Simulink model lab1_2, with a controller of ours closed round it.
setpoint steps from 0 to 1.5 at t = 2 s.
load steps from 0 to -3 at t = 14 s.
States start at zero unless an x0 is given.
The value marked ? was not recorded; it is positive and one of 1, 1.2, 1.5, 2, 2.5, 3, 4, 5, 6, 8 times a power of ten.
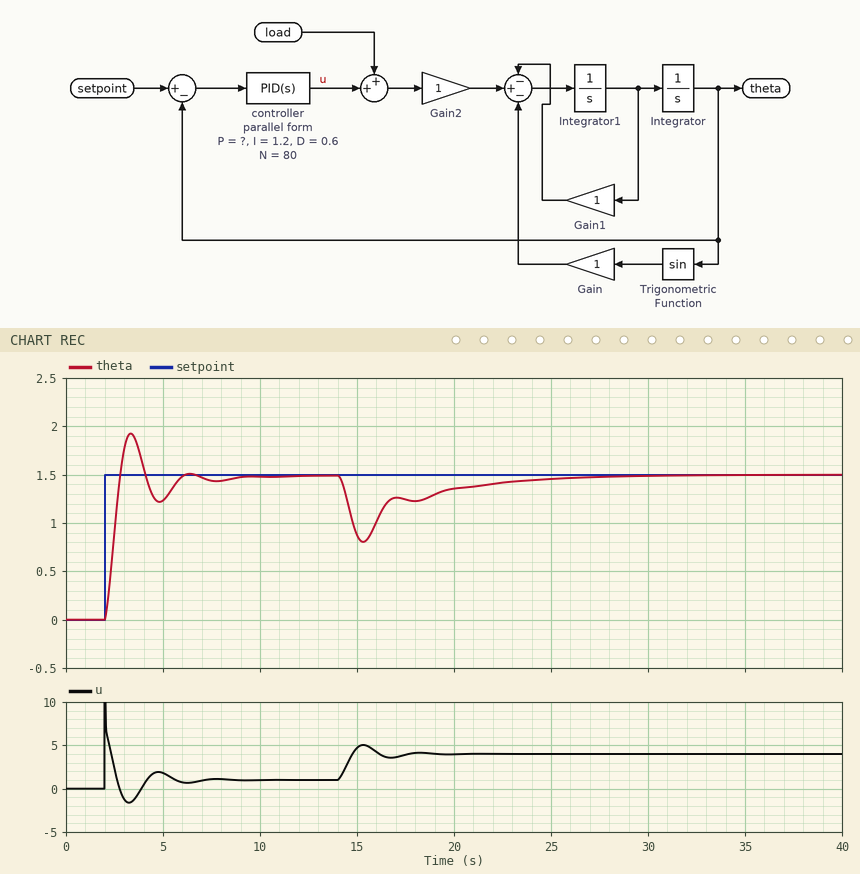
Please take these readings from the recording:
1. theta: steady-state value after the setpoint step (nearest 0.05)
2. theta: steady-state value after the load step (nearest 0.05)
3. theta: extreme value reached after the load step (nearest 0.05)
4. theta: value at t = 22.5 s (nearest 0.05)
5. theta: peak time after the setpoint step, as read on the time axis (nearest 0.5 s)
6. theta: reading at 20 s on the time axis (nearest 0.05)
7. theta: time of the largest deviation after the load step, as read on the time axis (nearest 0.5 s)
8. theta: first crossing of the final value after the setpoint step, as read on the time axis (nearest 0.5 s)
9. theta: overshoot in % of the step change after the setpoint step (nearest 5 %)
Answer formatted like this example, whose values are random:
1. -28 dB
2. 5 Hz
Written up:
1. 1.50
2. 1.50
3. 0.80
4. 1.40
5. 3.5 s
6. 1.35
7. 15.5 s
8. 3.0 s
9. 30 %
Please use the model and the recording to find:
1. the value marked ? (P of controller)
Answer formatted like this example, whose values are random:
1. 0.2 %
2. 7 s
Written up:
1. 5
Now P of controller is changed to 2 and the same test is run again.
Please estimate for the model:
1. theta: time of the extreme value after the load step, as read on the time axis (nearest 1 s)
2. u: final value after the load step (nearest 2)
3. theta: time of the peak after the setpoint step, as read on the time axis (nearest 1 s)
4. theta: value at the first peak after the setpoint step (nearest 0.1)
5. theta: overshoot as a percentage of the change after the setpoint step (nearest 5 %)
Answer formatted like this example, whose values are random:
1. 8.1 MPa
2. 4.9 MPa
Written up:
1. 16 s
2. 4
3. 4 s
4. 1.8
5. 20 %
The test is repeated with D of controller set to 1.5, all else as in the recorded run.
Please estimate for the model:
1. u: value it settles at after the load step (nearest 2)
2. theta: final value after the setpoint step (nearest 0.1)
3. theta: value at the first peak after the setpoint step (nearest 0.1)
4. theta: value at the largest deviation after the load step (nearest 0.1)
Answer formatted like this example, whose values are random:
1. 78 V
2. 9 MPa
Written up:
1. 4
2. 1.5
3. 1.7
4. 0.9
